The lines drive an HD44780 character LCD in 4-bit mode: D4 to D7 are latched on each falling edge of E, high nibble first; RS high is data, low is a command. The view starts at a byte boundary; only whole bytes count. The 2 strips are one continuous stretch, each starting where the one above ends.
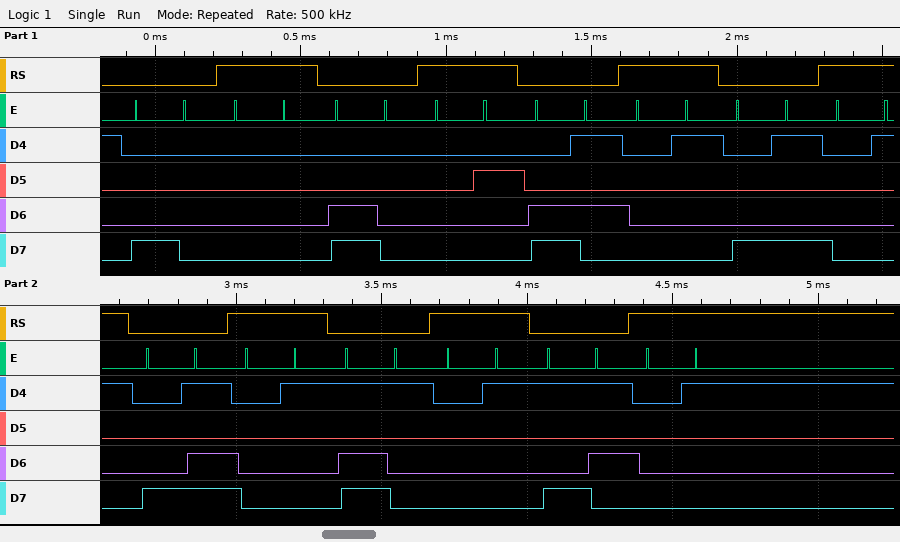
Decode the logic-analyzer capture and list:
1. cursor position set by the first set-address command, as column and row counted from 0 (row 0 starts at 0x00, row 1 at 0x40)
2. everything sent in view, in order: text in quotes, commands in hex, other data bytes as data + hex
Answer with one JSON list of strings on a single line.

["column 0, row 0", "0x80 data 00 0xC0 data 02 0xC5 data 01 0x89 data 01 0x8D data 01 0xD1 data 01 0x95 data 01"]
